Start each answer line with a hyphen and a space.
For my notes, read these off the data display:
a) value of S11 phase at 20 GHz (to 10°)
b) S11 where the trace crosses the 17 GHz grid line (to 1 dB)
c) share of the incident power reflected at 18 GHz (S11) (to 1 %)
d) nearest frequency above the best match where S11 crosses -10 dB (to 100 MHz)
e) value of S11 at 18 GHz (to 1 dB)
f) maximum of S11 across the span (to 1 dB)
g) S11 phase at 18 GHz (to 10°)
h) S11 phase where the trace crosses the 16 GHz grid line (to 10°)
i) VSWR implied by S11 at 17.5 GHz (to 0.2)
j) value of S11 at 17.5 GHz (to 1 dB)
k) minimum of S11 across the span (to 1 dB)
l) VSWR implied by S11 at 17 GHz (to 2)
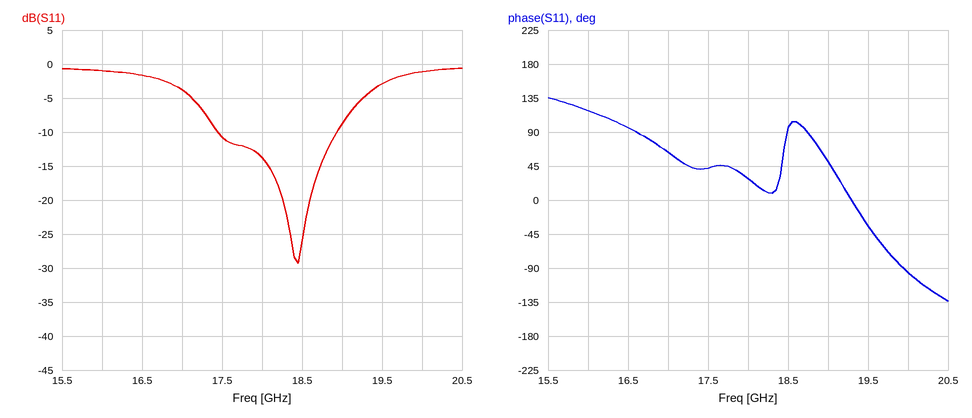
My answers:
- -100°
- -4 dB
- 4 %
- 18.9 GHz
- -14 dB
- -1 dB
- 30°
- 120°
- 1.8
- -11 dB
- -29 dB
- 4
